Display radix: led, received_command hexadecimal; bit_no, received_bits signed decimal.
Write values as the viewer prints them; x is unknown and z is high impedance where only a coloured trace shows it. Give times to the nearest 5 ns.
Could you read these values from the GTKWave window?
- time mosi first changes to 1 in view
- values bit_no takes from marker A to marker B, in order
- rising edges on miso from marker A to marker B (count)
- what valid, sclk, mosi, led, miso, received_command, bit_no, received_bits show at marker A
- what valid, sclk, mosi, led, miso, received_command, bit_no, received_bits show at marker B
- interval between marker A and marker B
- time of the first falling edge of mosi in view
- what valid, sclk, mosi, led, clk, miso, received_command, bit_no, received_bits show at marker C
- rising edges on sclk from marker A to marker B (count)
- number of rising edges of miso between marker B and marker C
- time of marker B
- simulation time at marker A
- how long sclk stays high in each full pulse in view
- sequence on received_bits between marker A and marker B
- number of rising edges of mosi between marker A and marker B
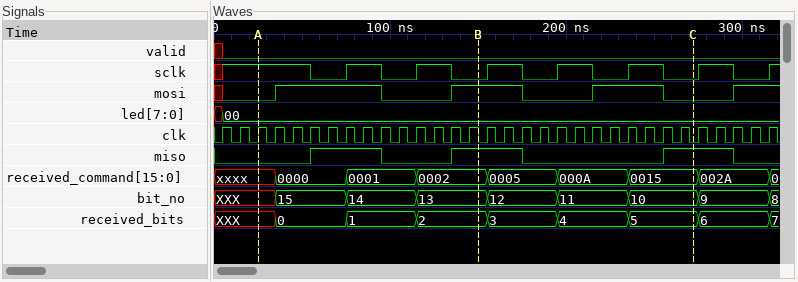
35 ns
XXX, 15, 14, 13
2
valid=0, sclk=1, mosi=0, led=00, miso=0, received_command=xxxx, bit_no=XXX, received_bits=XXX
valid=0, sclk=0, mosi=1, led=00, miso=1, received_command=0002, bit_no=13, received_bits=2
125 ns
95 ns
valid=0, sclk=0, mosi=0, led=00, clk=0, miso=1, received_command=0015, bit_no=10, received_bits=5
2
1
150 ns
25 ns
20 ns, 20 ns, 20 ns, 20 ns, 20 ns, 20 ns
XXX, 0, 1, 2
2
